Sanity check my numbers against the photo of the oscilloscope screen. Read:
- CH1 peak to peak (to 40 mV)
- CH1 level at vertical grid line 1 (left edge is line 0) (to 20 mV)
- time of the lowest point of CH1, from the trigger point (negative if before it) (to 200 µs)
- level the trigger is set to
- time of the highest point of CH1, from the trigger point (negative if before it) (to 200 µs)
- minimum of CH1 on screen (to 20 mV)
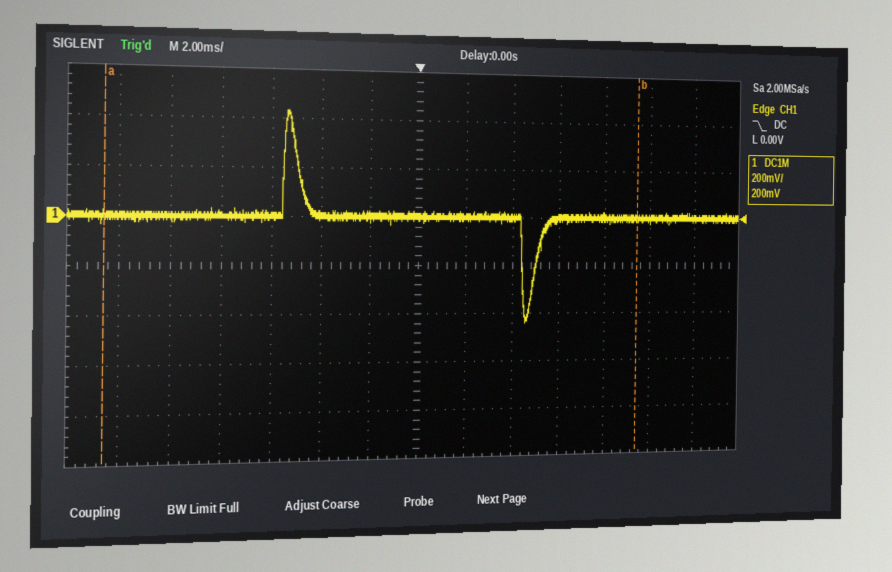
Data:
880 mV
0 mV
+4.6 ms
0.00 V
-5.4 ms
-440 mV
